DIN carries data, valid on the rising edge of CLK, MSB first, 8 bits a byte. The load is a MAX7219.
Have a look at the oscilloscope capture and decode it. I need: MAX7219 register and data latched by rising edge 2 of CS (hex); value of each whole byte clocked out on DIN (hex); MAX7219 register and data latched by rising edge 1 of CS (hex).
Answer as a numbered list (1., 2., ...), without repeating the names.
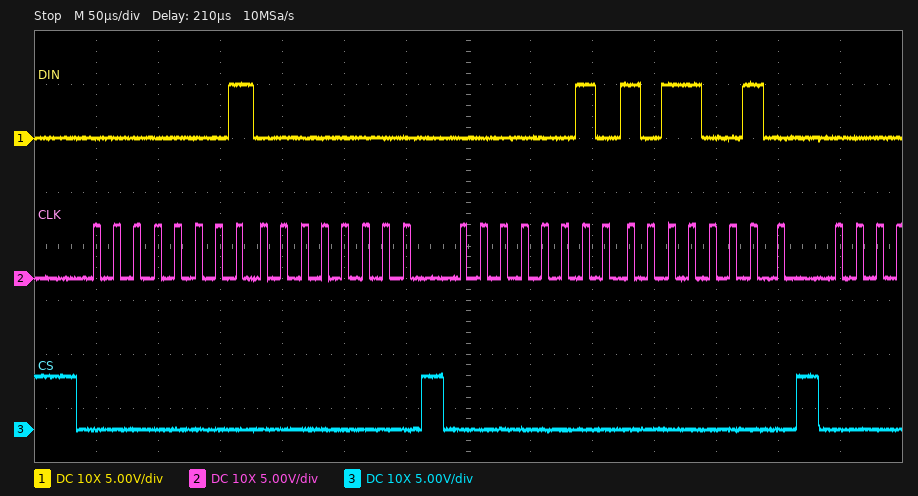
1. register 0x2, data 0xB2
2. 01 00 02 B2
3. register 0x1, data 0x00
